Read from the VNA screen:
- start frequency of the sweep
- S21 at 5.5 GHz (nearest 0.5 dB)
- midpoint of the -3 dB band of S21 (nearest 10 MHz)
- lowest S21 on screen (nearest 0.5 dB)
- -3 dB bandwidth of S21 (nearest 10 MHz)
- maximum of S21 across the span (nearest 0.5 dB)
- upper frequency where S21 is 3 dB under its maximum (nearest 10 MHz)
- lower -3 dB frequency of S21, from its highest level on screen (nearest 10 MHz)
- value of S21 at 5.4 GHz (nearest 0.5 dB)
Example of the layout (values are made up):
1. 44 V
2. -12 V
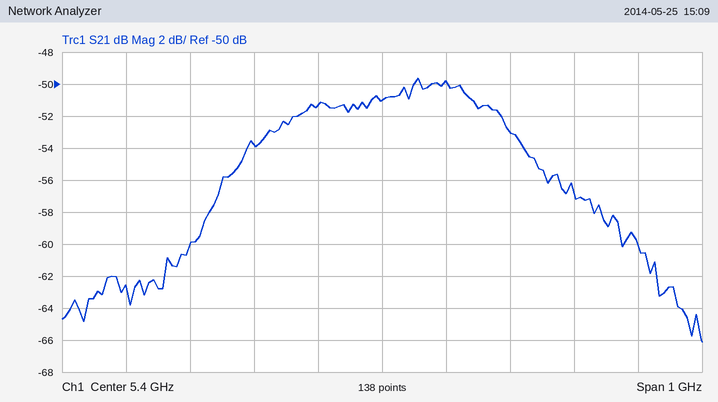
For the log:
1. 4.9 GHz
2. -50.0 dB
3. 5.42 GHz
4. -66.0 dB
5. 350 MHz
6. -49.5 dB
7. 5.59 GHz
8. 5.24 GHz
9. -51.0 dB
